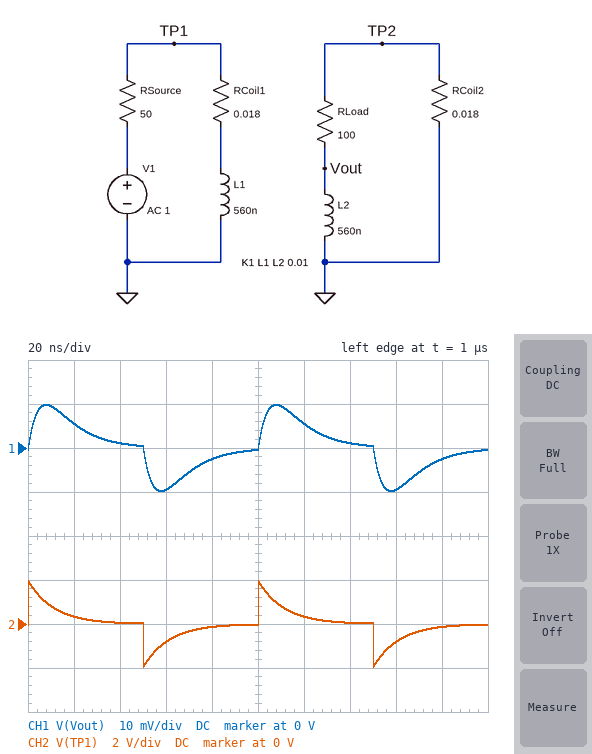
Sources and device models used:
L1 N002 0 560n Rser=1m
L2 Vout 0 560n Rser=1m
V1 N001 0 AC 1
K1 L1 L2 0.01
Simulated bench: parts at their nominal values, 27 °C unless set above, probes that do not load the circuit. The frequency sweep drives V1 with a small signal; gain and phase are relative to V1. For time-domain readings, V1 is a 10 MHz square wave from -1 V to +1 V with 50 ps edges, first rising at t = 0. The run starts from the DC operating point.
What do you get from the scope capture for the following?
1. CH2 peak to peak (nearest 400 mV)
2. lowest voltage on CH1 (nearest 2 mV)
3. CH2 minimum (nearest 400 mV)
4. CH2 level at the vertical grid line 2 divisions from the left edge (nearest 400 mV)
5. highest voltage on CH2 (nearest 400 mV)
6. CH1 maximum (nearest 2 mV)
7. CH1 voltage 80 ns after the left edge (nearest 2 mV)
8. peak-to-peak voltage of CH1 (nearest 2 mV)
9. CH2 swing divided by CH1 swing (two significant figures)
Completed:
4.0 V
-10 mV
-2.0 V
0 V
2.0 V
10 mV
-2 mV
20 mV
200
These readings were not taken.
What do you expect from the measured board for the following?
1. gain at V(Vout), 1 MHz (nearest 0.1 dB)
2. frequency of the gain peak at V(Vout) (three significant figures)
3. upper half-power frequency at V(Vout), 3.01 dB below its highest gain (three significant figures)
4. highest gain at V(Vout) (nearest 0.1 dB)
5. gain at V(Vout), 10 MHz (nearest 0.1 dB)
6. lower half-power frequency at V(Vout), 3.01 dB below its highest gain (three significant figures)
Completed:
-63.1 dB
20.1 MHz
50.6 MHz
-43.5 dB
-45.3 dB
7.98 MHz
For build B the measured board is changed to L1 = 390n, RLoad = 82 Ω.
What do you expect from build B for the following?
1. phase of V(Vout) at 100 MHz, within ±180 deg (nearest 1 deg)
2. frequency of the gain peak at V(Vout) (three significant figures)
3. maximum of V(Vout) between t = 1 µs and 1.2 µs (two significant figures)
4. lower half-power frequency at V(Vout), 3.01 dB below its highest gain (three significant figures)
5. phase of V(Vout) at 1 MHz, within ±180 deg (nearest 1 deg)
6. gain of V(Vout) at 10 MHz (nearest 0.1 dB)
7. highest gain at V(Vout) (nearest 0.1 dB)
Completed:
-65 deg
21.8 MHz
9.3 mV
9.02 MHz
85 deg
-46.3 dB
-43.9 dB
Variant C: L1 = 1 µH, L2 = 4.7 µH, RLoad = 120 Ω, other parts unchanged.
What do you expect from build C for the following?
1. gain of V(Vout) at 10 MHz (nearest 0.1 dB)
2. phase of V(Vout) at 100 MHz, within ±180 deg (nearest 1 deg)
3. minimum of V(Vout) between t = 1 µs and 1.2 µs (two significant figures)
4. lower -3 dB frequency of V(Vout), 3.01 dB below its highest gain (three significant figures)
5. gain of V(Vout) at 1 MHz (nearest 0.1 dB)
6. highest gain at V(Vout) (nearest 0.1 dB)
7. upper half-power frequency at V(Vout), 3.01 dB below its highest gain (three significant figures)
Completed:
-43.9 dB
-83 deg
-7.2 mV
2.26 MHz
-51.6 dB
-42.7 dB
14.3 MHz
